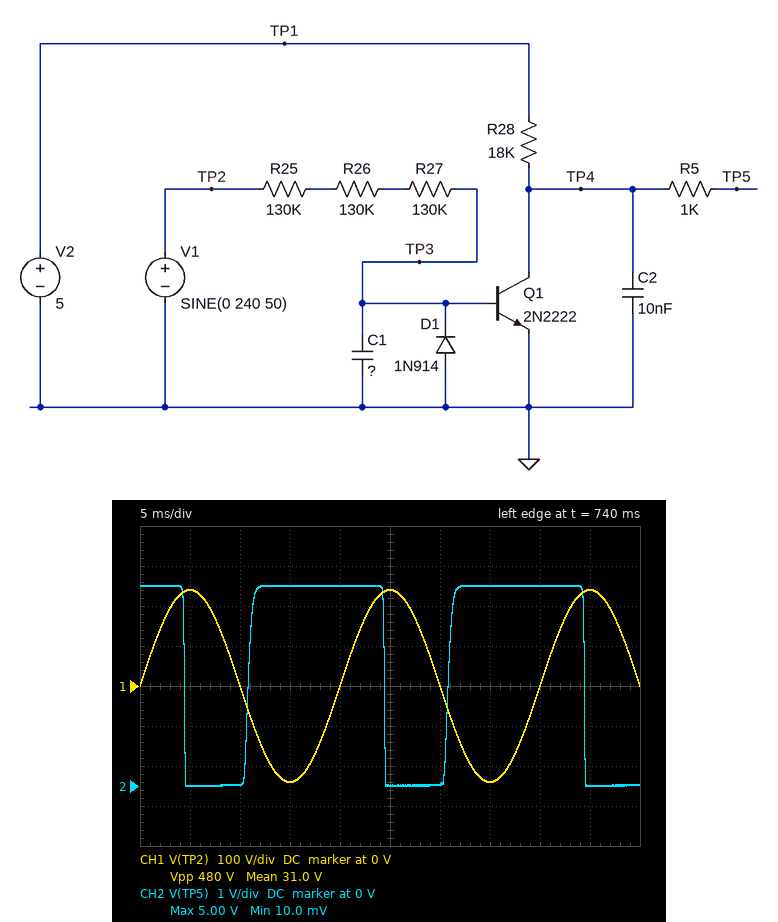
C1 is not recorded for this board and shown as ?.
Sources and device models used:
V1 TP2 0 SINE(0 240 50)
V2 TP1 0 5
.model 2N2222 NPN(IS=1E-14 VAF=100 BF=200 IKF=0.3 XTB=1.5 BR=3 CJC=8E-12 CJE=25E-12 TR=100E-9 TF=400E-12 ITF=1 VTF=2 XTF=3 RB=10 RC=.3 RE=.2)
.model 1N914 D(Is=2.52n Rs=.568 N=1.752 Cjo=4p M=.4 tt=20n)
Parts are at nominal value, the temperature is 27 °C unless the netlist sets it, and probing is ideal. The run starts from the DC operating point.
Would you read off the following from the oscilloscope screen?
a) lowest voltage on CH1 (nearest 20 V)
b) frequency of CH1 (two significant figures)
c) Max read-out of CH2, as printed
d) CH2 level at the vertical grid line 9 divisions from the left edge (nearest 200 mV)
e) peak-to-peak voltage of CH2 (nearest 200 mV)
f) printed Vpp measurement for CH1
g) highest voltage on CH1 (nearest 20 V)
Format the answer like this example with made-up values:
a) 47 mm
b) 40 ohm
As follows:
a) -240 V
b) 50 Hz
c) 5.00 V
d) 0 V
e) 5.0 V
f) 480 V
g) 240 V
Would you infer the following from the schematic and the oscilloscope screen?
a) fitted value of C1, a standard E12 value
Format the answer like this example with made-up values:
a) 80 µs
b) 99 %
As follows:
a) 1.5 µF
